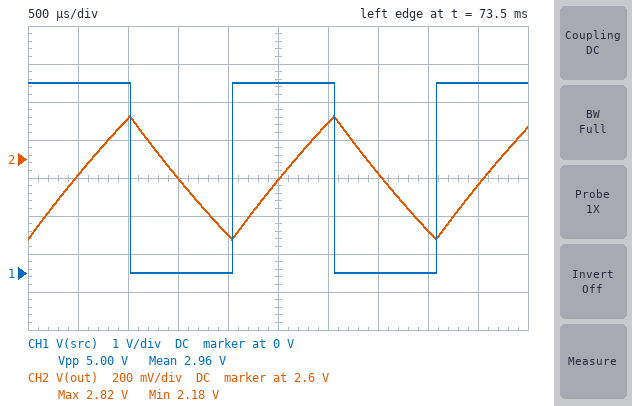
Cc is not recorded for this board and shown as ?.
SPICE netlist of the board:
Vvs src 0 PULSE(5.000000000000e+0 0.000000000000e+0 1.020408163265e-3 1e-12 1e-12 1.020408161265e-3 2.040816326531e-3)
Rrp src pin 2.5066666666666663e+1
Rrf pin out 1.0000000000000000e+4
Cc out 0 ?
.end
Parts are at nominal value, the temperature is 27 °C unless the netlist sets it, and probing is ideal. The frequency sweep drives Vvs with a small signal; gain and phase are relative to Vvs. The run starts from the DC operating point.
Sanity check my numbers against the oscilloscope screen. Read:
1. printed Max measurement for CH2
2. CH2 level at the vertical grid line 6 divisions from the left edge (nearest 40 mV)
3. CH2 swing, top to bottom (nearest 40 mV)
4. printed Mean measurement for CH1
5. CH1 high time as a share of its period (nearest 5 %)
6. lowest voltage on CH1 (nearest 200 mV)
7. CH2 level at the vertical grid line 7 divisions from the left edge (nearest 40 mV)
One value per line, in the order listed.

2.82 V
2.80 V
640 mV
2.96 V
50 %
0 V
2.52 V
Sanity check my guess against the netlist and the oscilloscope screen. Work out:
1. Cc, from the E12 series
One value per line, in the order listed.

390 nF
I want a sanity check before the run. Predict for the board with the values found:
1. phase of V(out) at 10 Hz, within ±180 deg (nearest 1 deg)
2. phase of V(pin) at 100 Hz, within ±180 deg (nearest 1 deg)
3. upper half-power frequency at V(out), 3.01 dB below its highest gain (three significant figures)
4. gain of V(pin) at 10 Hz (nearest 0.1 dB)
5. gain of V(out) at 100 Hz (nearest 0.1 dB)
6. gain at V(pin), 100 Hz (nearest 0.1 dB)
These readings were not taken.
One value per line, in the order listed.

-14 deg
0 deg
40.7 Hz
0 dB
-8.5 dB
0 dB
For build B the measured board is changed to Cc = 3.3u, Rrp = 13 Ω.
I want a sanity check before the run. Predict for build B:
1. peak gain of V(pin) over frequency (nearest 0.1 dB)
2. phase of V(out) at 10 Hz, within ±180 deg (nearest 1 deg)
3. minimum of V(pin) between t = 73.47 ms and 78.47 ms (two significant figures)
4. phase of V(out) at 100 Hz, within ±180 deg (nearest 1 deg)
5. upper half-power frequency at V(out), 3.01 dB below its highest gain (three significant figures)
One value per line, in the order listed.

0 dB
-64 deg
3.5 mV
-87 deg
4.82 Hz
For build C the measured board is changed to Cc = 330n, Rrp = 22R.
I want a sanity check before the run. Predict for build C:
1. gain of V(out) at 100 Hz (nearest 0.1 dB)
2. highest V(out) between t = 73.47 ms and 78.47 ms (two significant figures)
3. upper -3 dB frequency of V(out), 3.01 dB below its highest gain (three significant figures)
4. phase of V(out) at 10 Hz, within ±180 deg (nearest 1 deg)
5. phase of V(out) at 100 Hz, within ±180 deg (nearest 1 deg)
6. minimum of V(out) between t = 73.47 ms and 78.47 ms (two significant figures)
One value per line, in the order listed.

-7.3 dB
2.9 V
48.1 Hz
-12 deg
-64 deg
2.1 V
